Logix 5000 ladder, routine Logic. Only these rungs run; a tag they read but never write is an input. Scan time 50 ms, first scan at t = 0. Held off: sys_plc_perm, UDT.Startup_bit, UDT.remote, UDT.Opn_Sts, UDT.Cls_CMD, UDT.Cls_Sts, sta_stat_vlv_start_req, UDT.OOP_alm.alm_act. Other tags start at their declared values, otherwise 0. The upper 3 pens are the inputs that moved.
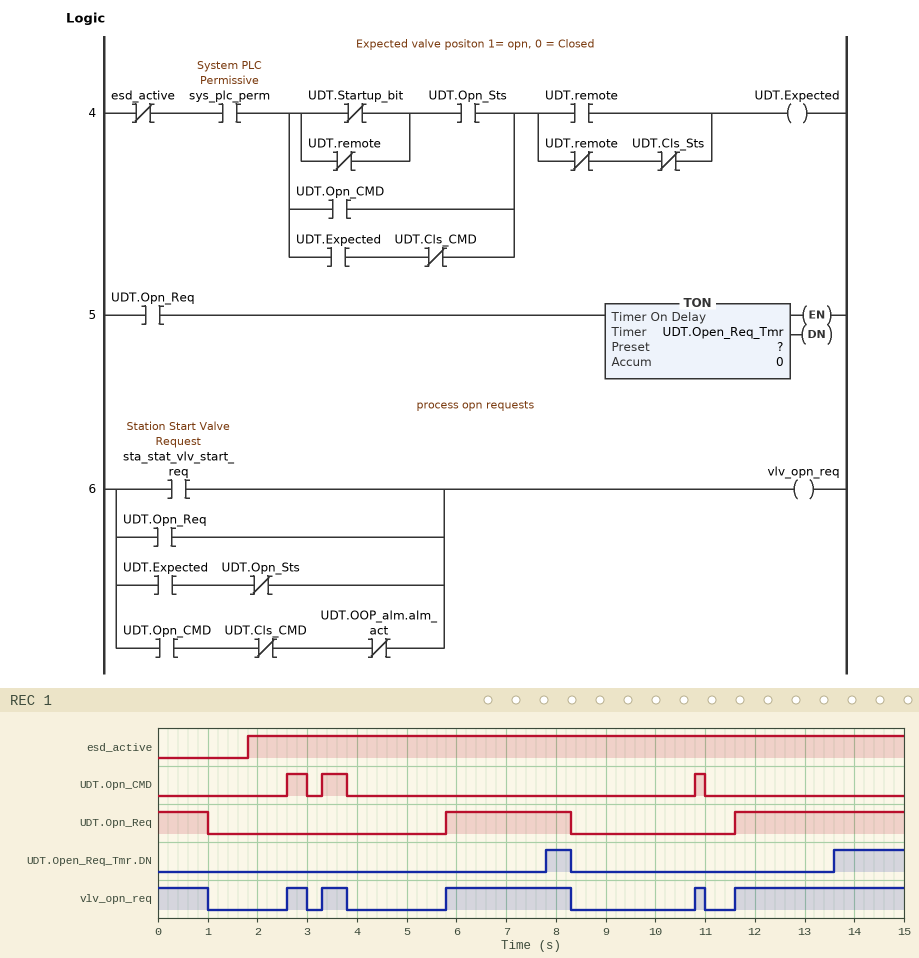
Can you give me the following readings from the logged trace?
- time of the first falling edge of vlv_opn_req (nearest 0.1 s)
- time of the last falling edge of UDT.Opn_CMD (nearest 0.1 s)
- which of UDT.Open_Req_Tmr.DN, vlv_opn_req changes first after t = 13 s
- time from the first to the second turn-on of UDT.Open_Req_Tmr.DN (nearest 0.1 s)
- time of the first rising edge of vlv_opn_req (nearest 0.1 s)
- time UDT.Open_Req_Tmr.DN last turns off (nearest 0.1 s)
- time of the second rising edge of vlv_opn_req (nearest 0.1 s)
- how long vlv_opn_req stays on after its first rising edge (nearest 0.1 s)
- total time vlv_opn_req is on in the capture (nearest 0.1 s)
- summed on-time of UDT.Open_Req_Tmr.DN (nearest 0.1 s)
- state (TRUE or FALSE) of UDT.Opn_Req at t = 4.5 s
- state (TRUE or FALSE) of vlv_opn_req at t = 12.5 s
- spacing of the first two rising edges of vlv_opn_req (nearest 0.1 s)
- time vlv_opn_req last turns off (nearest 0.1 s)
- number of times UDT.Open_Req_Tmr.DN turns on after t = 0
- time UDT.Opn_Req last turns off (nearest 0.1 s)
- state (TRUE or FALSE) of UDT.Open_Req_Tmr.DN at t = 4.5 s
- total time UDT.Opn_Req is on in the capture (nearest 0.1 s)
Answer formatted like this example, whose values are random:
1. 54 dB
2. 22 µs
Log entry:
1. 1.0 s
2. 11.0 s
3. UDT.Open_Req_Tmr.DN
4. 5.8 s
5. 2.6 s
6. 8.3 s
7. 3.3 s
8. 0.4 s
9. 8.0 s
10. 1.9 s
11. FALSE
12. TRUE
13. 0.7 s
14. 11.0 s
15. 2
16. 8.3 s
17. FALSE
18. 6.9 s
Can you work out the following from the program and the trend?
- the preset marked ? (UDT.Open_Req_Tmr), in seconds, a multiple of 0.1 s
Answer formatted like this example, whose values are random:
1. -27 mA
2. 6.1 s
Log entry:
1. 2.0 s
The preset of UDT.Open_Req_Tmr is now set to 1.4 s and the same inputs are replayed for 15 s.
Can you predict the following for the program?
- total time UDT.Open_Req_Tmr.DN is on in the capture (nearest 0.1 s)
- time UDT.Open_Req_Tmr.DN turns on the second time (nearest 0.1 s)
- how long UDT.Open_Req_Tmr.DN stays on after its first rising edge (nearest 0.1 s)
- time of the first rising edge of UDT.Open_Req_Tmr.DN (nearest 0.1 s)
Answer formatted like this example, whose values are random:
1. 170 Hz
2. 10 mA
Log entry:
1. 3.1 s
2. 13.0 s
3. 1.1 s
4. 7.2 s
